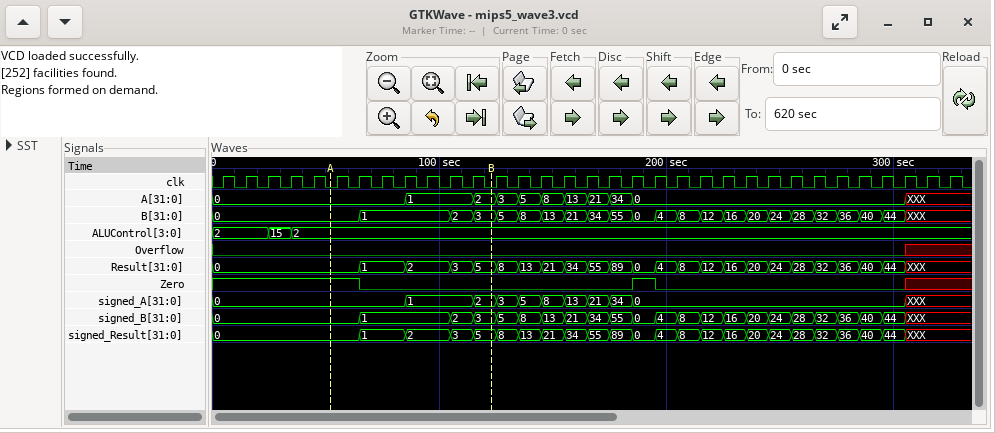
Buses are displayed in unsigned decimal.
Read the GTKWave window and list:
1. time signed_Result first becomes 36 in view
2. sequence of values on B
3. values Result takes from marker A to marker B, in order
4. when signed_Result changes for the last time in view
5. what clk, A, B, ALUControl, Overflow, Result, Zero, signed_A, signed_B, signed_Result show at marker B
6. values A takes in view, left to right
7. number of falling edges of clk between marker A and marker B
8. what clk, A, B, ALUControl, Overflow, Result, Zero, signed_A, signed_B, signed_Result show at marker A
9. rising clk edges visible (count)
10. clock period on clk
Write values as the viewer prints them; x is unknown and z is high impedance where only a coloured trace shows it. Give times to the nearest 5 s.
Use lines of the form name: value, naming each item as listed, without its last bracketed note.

time signed_Result first becomes 36 in view: 275 s
sequence of values on B: 0, 1, 2, 3, 5, 8, 13, 21, 34, 55, 0, 4, 8, 12, 16, 20, 24, 28, 32, 36, 40, 44, XXX
values Result takes from marker A to marker B, in order: 0, 1, 2, 3, 5
when signed_Result changes for the last time in view: 305 s
what clk, A, B, ALUControl, Overflow, Result, Zero, signed_A, signed_B, signed_Result show at marker B: clk=0, A=2, B=3, ALUControl=2, Overflow=0, Result=5, Zero=0, signed_A=2, signed_B=3, signed_Result=5
values A takes in view, left to right: 0, 1, 2, 3, 5, 8, 13, 21, 34, 0, XXX
number of falling edges of clk between marker A and marker B: 7
what clk, A, B, ALUControl, Overflow, Result, Zero, signed_A, signed_B, signed_Result show at marker A: clk=0, A=0, B=0, ALUControl=2, Overflow=0, Result=0, Zero=1, signed_A=0, signed_B=0, signed_Result=0
rising clk edges visible: 33
clock period on clk: 10 s
